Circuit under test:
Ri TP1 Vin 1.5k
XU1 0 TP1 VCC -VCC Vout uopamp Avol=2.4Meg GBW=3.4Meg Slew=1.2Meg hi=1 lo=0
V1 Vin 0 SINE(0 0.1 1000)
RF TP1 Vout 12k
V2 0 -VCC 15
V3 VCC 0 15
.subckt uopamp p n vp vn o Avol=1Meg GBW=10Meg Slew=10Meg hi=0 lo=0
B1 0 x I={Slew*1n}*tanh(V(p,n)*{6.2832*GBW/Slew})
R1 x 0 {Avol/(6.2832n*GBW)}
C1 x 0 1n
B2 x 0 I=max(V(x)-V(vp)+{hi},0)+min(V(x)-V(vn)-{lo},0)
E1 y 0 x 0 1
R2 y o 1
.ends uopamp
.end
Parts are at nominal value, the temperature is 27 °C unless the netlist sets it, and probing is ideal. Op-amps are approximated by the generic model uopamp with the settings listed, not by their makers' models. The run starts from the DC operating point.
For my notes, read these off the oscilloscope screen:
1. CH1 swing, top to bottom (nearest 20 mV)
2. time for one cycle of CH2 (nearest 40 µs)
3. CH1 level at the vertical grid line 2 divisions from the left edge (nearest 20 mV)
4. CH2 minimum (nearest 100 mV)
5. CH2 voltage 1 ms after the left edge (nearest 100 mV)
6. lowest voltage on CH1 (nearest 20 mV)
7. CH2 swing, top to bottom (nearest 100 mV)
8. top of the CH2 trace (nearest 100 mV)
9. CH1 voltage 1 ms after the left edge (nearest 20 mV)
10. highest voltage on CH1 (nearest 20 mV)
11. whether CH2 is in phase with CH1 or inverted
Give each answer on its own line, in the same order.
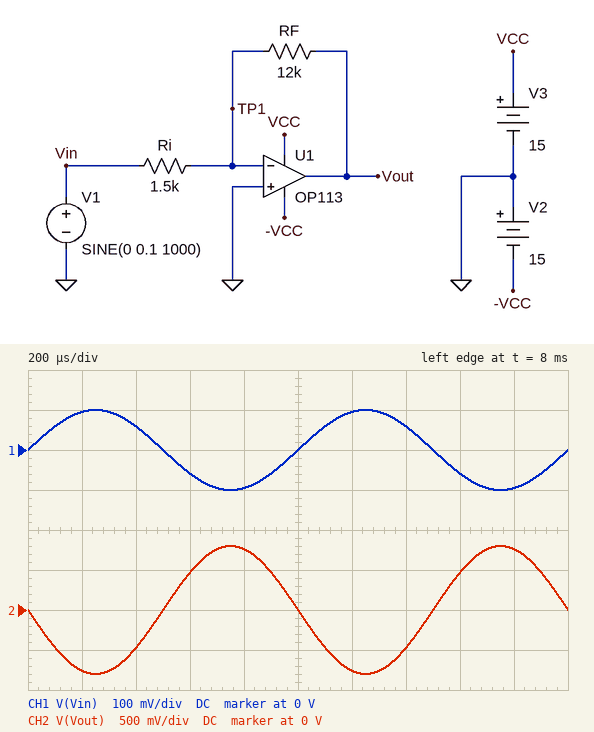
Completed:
200 mV
1.00 ms
60 mV
-800 mV
0 V
-100 mV
1.6 V
800 mV
0 V
100 mV
inverted
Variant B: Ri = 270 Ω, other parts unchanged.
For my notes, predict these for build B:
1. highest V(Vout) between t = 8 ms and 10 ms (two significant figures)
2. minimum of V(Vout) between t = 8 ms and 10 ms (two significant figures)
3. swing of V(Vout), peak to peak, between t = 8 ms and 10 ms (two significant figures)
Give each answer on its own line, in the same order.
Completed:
4.4 V
-4.4 V
8.9 V
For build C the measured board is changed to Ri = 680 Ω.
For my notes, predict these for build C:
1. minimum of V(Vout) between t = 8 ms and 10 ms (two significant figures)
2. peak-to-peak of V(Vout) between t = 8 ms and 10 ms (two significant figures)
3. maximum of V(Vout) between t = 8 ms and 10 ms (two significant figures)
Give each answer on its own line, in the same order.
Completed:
-1.8 V
3.5 V
1.8 V
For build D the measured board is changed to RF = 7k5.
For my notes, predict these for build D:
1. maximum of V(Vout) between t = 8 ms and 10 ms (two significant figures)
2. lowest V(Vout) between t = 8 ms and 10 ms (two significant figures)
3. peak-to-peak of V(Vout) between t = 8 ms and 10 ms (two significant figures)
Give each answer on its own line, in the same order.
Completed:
500 mV
-500 mV
1.0 V
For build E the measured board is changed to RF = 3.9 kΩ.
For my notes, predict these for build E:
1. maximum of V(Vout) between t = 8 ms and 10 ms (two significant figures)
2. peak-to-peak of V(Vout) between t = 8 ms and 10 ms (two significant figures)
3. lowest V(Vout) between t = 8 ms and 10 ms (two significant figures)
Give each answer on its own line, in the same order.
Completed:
260 mV
520 mV
-260 mV
